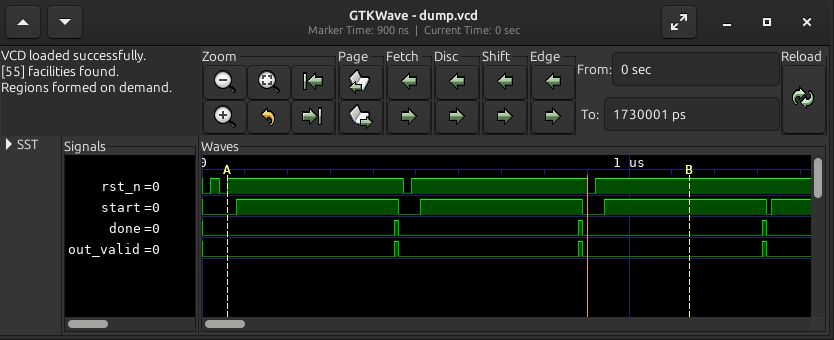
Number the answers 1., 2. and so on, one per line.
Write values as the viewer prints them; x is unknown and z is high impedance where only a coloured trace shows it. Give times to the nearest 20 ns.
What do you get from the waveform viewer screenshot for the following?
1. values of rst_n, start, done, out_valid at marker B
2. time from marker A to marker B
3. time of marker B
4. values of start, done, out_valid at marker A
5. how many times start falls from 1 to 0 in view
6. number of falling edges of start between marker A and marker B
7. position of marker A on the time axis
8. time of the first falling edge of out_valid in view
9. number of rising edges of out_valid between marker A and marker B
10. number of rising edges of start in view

1. rst_n=1, start=1, done=0, out_valid=0
2. 1080 ns
3. 1140 ns
4. start=0, done=0, out_valid=0
5. 3
6. 2
7. 60 ns
8. 460 ns
9. 2
10. 4
